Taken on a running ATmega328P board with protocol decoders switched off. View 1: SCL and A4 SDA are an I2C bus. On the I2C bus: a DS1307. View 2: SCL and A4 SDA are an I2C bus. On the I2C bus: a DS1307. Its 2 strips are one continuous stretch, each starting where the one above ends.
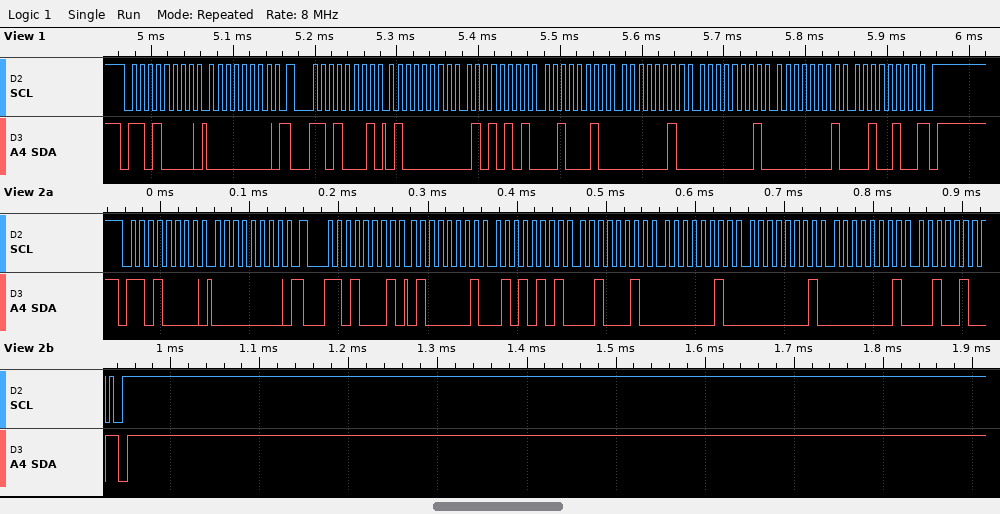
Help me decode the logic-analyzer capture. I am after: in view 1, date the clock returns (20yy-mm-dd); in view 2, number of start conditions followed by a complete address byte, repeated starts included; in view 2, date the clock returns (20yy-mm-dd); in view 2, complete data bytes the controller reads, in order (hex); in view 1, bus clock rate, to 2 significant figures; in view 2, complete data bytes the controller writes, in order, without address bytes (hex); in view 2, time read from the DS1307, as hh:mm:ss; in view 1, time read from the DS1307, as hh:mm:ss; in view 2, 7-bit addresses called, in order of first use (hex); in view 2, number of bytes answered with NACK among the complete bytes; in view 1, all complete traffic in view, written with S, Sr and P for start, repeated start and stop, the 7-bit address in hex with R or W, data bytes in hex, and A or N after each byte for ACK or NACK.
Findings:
2024-01-01
2
2024-01-01
41 55 22 02 01 01 24
100 kHz
00
22:55:41
22:55:40
0x68
1
S 68W A 00 A Sr 68R A 40 A 55 A 22 A 02 A 01 A 01 A 24 N P
